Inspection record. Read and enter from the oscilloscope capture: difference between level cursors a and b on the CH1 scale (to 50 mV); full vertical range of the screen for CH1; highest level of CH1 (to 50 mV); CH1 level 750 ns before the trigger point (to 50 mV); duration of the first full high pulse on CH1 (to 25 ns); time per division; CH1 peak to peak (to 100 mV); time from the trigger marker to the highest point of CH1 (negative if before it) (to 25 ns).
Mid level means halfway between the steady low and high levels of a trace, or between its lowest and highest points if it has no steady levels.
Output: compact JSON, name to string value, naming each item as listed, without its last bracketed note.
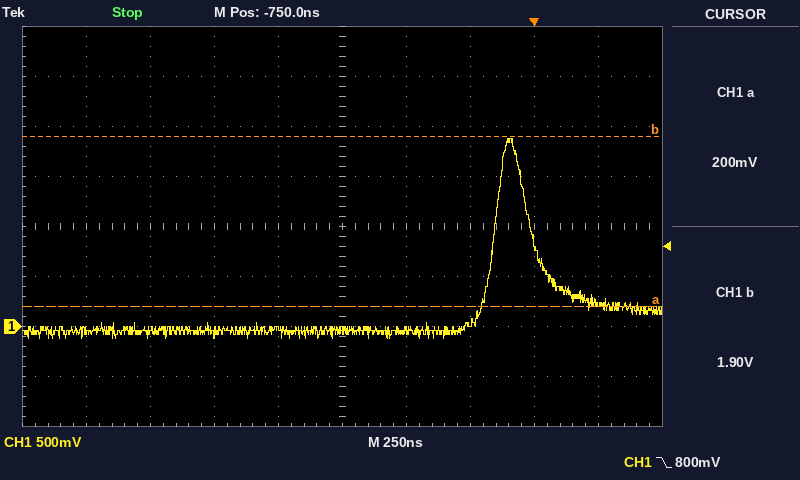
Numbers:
{"difference between level cursors a and b on the CH1 scale": "1.70 V", "full vertical range of the screen for CH1": "4 V", "highest level of CH1": "1.90 V", "CH1 level 750 ns before the trigger point": "-50 mV", "duration of the first full high pulse on CH1": "150 ns", "time per division": "250 ns", "CH1 peak to peak": "2.00 V", "time from the trigger marker to the highest point of CH1 (negative if before it)": "-100 ns"}
